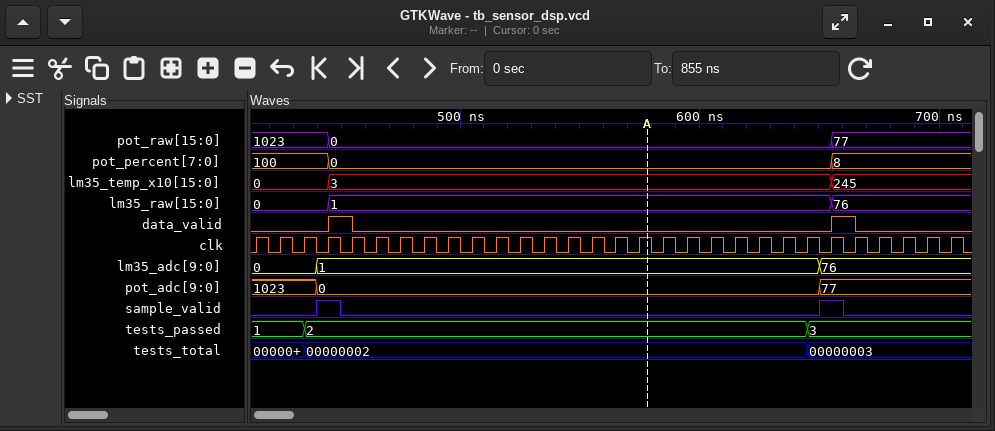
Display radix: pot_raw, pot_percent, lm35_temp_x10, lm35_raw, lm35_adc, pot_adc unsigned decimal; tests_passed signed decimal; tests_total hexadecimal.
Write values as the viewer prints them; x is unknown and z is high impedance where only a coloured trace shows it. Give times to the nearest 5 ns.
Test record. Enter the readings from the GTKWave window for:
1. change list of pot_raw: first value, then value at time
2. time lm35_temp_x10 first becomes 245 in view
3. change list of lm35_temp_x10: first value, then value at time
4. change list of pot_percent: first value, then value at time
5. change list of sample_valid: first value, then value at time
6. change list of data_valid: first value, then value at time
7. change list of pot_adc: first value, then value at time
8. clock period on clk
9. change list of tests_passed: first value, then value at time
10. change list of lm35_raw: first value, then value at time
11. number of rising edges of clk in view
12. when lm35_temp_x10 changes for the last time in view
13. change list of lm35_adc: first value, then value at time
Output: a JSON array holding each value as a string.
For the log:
["1023, 0 at 445 ns, 77 at 655 ns", "655 ns", "0, 3 at 445 ns, 245 at 655 ns", "100, 0 at 445 ns, 8 at 655 ns", "0, 1 at 440 ns, 0 at 450 ns, 1 at 650 ns, 0 at 660 ns", "0, 1 at 445 ns, 0 at 455 ns, 1 at 655 ns, 0 at 665 ns", "1023, 0 at 440 ns, 77 at 650 ns", "10 ns", "1, 2 at 435 ns, 3 at 645 ns", "0, 1 at 445 ns, 76 at 655 ns", "30", "655 ns", "0, 1 at 440 ns, 76 at 650 ns"]
